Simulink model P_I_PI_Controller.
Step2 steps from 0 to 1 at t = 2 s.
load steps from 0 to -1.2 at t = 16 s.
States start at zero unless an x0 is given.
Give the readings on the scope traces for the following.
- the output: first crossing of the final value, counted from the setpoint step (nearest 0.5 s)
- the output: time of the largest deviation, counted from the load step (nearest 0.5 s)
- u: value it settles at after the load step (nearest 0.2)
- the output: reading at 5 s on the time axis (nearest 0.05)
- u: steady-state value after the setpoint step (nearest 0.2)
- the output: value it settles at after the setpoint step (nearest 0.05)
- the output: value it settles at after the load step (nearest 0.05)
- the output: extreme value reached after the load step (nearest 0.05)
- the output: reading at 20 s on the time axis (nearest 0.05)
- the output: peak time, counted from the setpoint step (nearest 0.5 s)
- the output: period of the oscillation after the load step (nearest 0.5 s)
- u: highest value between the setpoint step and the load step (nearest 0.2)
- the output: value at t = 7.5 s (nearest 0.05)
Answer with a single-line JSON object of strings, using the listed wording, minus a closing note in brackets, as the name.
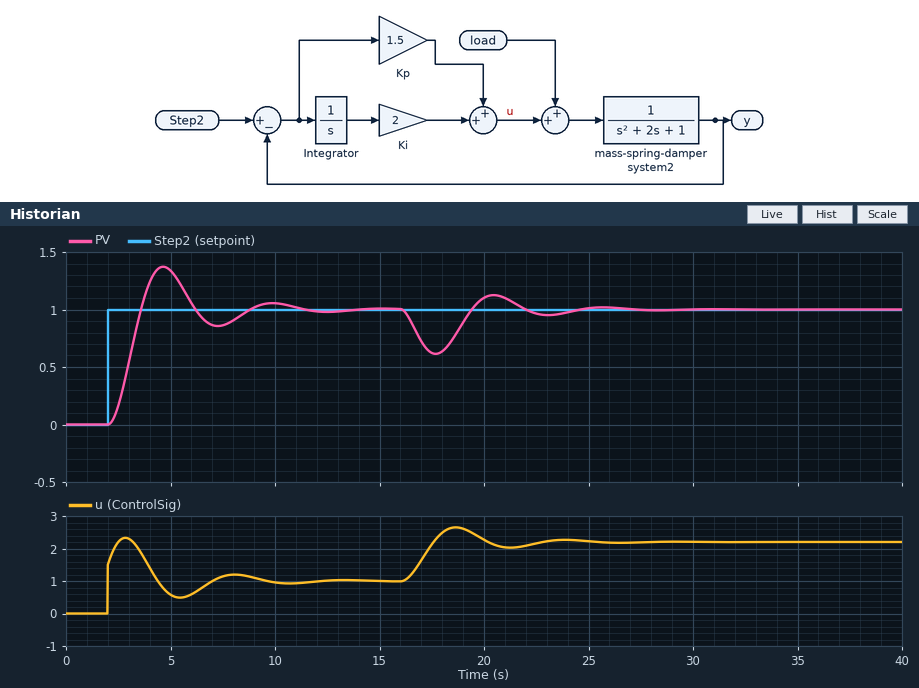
{"the output: first crossing of the final value, counted from the setpoint step": "1.5 s", "the output: time of the largest deviation, counted from the load step": "1.5 s", "u: value it settles at after the load step": "2.2", "the output: reading at 5 s on the time axis": "1.35", "u: steady-state value after the setpoint step": "1.0", "the output: value it settles at after the setpoint step": "1.00", "the output: value it settles at after the load step": "1.00", "the output: extreme value reached after the load step": "0.60", "the output: reading at 20 s on the time axis": "1.10", "the output: peak time, counted from the setpoint step": "2.5 s", "the output: period of the oscillation after the load step": "5.5 s", "u: highest value between the setpoint step and the load step": "2.4", "the output: value at t = 7.5 s": "0.85"}
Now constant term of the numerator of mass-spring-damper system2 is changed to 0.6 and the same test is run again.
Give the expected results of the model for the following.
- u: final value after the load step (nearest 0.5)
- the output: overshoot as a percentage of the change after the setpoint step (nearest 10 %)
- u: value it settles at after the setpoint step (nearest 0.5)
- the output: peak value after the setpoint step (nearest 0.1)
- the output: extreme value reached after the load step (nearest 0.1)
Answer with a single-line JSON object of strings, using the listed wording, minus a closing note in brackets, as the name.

{"u: final value after the load step": "3.0", "the output: overshoot as a percentage of the change after the setpoint step": "30 %", "u: value it settles at after the setpoint step": "1.5", "the output: peak value after the setpoint step": "1.3", "the output: extreme value reached after the load step": "0.7"}
